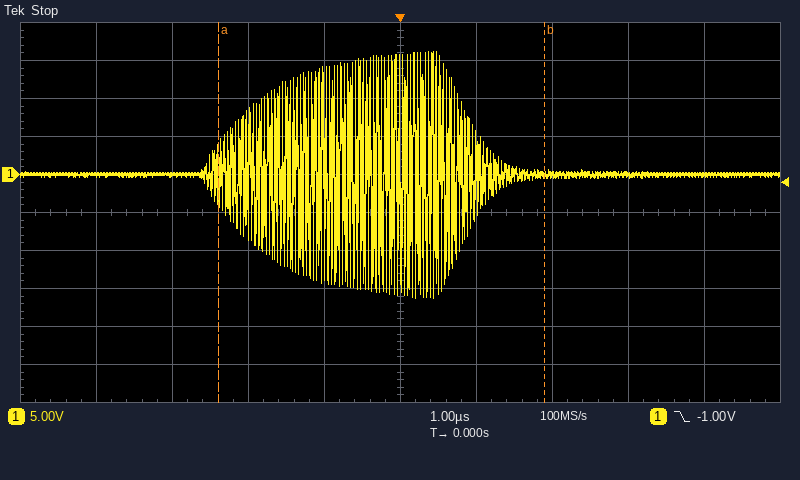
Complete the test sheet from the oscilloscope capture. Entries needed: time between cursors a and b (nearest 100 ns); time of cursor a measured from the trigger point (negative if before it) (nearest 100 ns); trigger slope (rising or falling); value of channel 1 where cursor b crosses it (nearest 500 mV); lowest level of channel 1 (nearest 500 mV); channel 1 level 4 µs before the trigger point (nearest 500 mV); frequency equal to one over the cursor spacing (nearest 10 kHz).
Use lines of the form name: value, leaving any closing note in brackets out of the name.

time between cursors a and b: 4.3 µs
time of cursor a measured from the trigger point (negative if before it): -2.4 µs
trigger slope: falling
value of channel 1 where cursor b crosses it: 0.0 V
lowest level of channel 1: -16.0 V
channel 1 level 4 µs before the trigger point: 0.0 V
frequency equal to one over the cursor spacing: 230 kHz
